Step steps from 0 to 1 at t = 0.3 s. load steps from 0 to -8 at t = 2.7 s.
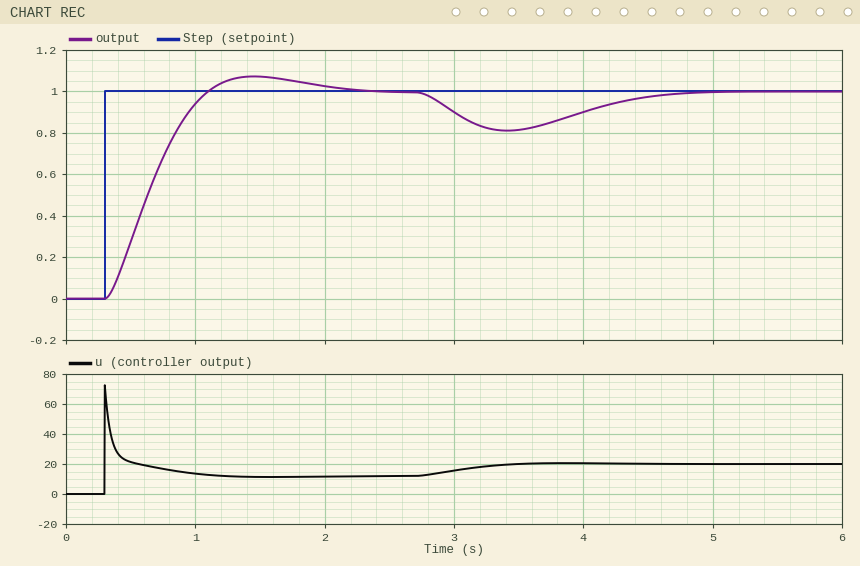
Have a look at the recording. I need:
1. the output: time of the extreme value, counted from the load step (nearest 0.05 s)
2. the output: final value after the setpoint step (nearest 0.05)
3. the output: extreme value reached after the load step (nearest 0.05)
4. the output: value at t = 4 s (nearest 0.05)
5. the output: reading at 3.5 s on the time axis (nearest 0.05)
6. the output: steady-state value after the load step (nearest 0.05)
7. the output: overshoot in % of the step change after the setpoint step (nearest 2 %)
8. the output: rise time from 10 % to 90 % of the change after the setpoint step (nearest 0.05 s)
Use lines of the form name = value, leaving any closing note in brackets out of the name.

the output: time of the extreme value, counted from the load step = 0.70 s
the output: final value after the setpoint step = 1.00
the output: extreme value reached after the load step = 0.80
the output: value at t = 4 s = 0.90
the output: reading at 3.5 s on the time axis = 0.80
the output: steady-state value after the load step = 1.00
the output: overshoot in % of the step change after the setpoint step = 8 %
the output: rise time from 10 % to 90 % of the change after the setpoint step = 0.55 s
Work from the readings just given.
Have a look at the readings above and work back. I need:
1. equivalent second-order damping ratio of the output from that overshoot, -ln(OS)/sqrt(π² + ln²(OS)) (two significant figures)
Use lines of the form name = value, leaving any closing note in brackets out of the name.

equivalent second-order damping ratio of the output from that overshoot, -ln(OS)/sqrt(π² + ln²(OS)) = 0.63
